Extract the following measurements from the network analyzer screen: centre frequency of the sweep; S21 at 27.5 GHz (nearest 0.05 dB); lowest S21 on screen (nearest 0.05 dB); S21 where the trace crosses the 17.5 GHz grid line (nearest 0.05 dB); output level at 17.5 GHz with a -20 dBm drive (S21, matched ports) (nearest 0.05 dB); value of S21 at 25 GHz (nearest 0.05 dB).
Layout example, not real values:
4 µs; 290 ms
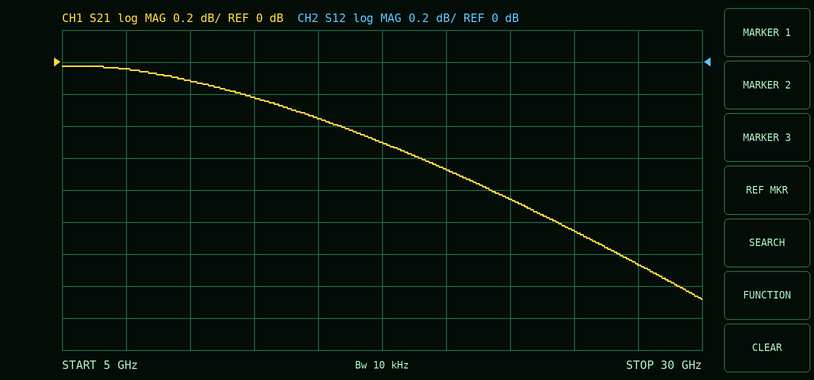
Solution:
17.5 GHz; -1.25 dB; -1.50 dB; -0.50 dB; -20.50 dBm; -1.05 dB
